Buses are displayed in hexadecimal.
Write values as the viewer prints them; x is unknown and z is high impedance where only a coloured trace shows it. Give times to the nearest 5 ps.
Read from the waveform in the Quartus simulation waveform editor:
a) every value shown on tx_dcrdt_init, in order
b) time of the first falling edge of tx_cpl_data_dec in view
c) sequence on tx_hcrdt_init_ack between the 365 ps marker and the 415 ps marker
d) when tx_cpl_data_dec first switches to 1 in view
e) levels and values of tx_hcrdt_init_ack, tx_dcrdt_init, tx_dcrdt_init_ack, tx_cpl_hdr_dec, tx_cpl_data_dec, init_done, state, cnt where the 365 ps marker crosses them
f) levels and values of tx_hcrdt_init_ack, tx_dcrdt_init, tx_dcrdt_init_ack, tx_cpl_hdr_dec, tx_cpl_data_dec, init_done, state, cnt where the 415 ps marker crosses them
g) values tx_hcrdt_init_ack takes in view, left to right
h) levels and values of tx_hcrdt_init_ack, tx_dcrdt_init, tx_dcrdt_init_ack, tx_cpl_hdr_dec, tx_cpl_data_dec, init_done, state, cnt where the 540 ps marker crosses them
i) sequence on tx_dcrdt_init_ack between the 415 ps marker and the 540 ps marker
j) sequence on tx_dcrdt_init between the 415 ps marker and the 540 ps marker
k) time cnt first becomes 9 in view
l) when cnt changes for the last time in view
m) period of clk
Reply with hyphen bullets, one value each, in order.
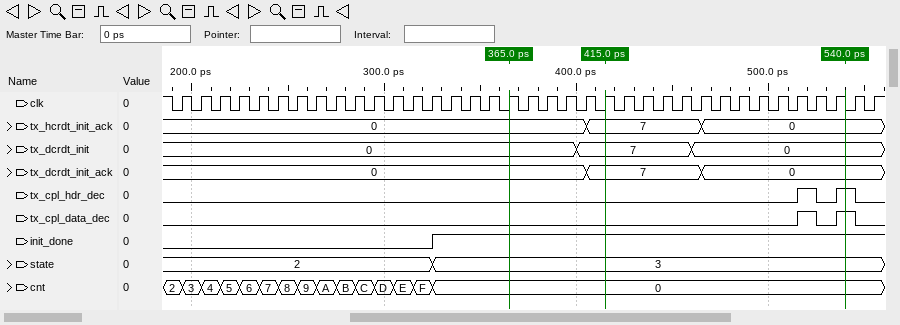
- 0, 7, 0
- 525 ps
- 0, 7
- 515 ps
- tx_hcrdt_init_ack=0, tx_dcrdt_init=0, tx_dcrdt_init_ack=0, tx_cpl_hdr_dec=0, tx_cpl_data_dec=0, init_done=1, state=3, cnt=0
- tx_hcrdt_init_ack=7, tx_dcrdt_init=7, tx_dcrdt_init_ack=7, tx_cpl_hdr_dec=0, tx_cpl_data_dec=0, init_done=1, state=3, cnt=0
- 0, 7, 0
- tx_hcrdt_init_ack=0, tx_dcrdt_init=0, tx_dcrdt_init_ack=0, tx_cpl_hdr_dec=1, tx_cpl_data_dec=1, init_done=1, state=3, cnt=0
- 7, 0
- 7, 0
- 255 ps
- 325 ps
- 10 ps
